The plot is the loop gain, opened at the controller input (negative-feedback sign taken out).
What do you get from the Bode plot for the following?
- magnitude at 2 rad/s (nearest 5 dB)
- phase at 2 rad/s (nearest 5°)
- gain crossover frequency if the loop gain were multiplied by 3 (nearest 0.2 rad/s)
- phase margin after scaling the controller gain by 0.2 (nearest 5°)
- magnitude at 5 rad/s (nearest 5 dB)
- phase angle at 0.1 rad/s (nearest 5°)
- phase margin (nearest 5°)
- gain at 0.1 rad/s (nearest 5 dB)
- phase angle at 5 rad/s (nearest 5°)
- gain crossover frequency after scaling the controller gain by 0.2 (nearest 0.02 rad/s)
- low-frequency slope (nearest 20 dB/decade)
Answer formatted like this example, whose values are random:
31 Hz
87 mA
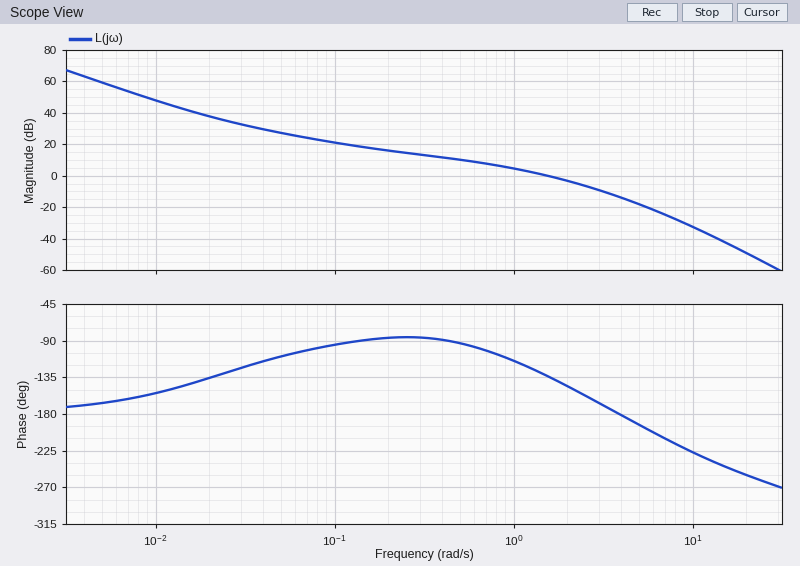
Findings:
-5 dB
-145°
3.0 rad/s
95°
-20 dB
-95°
45°
20 dB
-195°
0.28 rad/s
-40 dB/decade
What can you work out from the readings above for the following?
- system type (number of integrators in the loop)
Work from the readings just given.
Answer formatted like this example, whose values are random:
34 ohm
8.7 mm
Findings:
2
